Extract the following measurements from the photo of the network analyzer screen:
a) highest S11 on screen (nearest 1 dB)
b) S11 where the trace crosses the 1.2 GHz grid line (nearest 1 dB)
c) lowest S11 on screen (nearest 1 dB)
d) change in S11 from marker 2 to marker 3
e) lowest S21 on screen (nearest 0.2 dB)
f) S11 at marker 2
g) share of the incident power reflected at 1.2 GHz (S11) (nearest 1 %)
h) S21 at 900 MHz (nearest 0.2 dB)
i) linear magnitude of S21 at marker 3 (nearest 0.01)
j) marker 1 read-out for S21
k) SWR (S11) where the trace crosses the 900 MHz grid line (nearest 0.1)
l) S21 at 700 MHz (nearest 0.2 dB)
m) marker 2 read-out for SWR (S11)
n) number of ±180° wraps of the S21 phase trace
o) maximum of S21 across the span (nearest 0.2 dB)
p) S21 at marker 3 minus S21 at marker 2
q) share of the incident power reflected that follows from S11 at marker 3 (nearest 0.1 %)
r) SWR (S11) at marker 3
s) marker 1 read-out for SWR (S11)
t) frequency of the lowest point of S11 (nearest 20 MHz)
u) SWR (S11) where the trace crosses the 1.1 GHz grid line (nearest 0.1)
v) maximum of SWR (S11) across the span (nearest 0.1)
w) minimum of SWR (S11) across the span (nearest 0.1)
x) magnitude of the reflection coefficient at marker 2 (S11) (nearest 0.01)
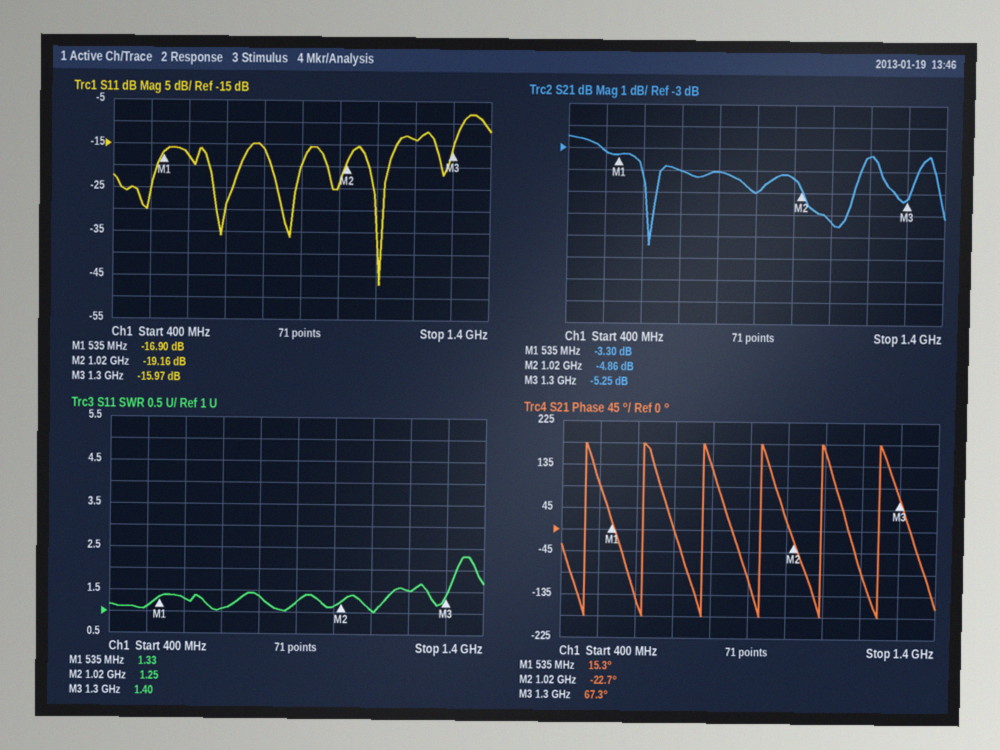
-8 dB
-14 dB
-47 dB
3.19 dB
-7.4 dB
-19.16 dB
4 %
-5.0 dB
0.55
-3.30 dB
1.2
-4.0 dB
1.25
6
-2.4 dB
-0.39 dB
2.5 %
1.40
1.33
1.10 GHz
1.1
2.3
1.0
0.11
